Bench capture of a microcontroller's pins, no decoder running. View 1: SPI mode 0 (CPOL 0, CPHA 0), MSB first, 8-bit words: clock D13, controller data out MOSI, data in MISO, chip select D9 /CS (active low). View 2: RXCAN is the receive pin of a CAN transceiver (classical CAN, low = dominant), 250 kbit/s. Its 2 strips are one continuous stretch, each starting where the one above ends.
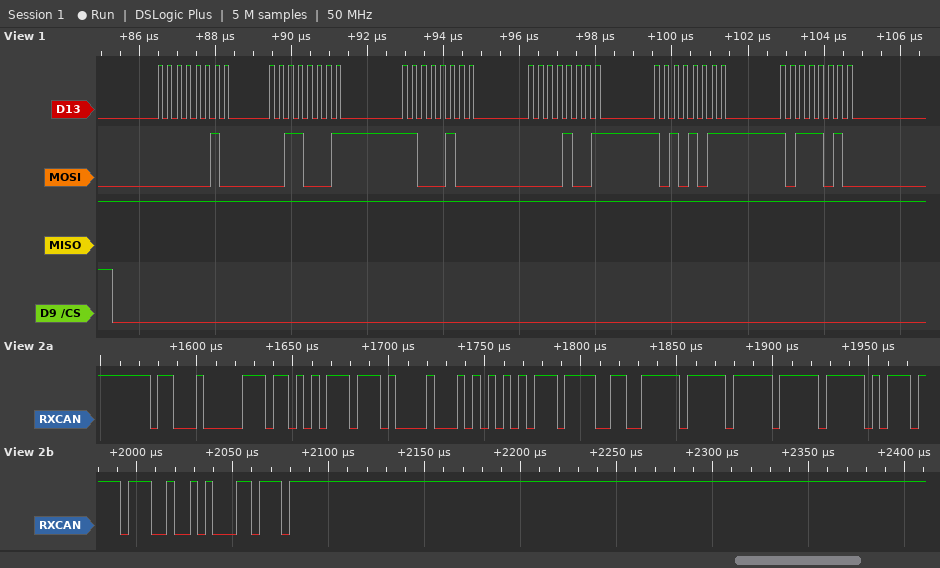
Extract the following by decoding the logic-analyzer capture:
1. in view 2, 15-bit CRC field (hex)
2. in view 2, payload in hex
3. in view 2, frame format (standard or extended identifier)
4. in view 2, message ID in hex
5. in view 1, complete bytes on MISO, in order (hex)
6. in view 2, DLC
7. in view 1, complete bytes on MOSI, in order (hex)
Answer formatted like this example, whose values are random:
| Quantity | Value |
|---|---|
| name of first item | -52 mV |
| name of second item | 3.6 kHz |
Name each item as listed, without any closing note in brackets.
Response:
| Quantity | Value |
|---|---|
| in view 2, 15-bit CRC field | 0x251B |
| in view 2, payload in hex | AA BB CC FF FF FF DD EE |
| in view 2, frame format | extended |
| in view 2, message ID in hex | 0x1881ABBA |
| in view 1, complete bytes on MISO, in order | FF FF FF FF FF FF |
| in view 2, DLC | 8 |
| in view 1, complete bytes on MOSI, in order | 02 31 C4 09 AB BA |
